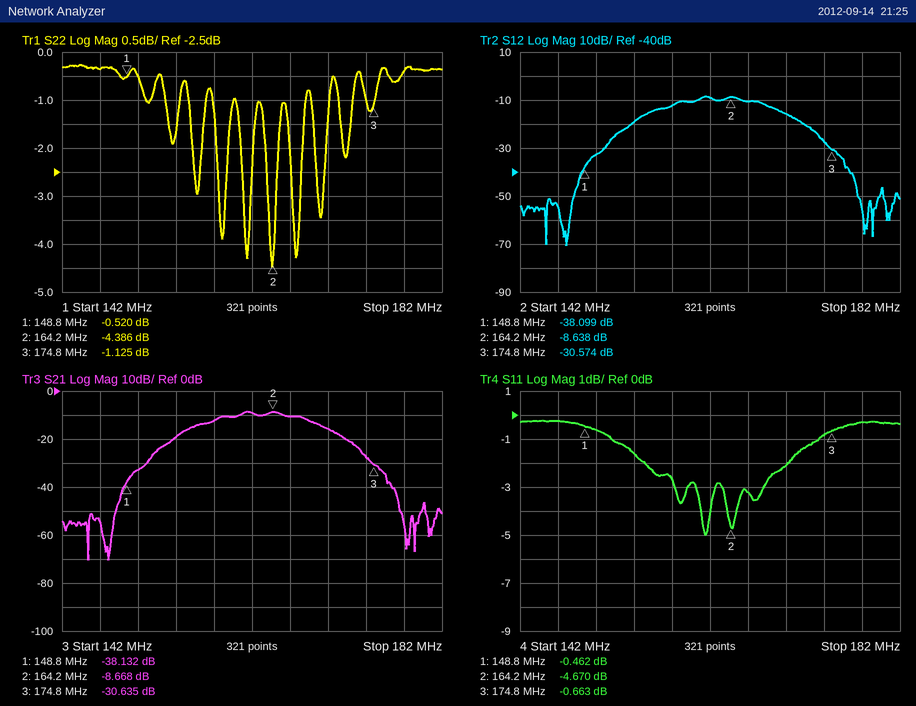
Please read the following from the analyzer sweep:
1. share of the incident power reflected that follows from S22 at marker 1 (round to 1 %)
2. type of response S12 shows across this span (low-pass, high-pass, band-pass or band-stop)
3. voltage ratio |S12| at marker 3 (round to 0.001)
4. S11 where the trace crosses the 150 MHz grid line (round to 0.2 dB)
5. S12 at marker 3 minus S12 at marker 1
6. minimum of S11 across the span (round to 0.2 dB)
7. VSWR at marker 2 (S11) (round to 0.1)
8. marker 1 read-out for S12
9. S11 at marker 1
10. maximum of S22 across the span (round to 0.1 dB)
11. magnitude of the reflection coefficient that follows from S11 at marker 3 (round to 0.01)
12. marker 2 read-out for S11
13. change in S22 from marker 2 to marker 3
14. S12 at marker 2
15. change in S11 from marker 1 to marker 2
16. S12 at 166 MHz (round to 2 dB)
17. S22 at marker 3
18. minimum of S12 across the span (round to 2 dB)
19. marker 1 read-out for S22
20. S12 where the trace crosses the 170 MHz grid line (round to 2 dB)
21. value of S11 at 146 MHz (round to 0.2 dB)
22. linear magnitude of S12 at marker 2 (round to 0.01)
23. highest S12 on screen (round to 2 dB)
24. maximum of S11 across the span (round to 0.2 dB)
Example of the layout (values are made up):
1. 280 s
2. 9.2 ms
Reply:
1. 89 %
2. band-pass
3. 0.030
4. -0.6 dB
5. 7.525 dB
6. -5.0 dB
7. 3.8
8. -38.099 dB
9. -0.462 dB
10. -0.3 dB
11. 0.93
12. -4.670 dB
13. 3.261 dB
14. -8.638 dB
15. -4.208 dB
16. -10 dB
17. -1.125 dB
18. -70 dB
19. -0.520 dB
20. -16 dB
21. -0.2 dB
22. 0.37
23. -8 dB
24. -0.2 dB
